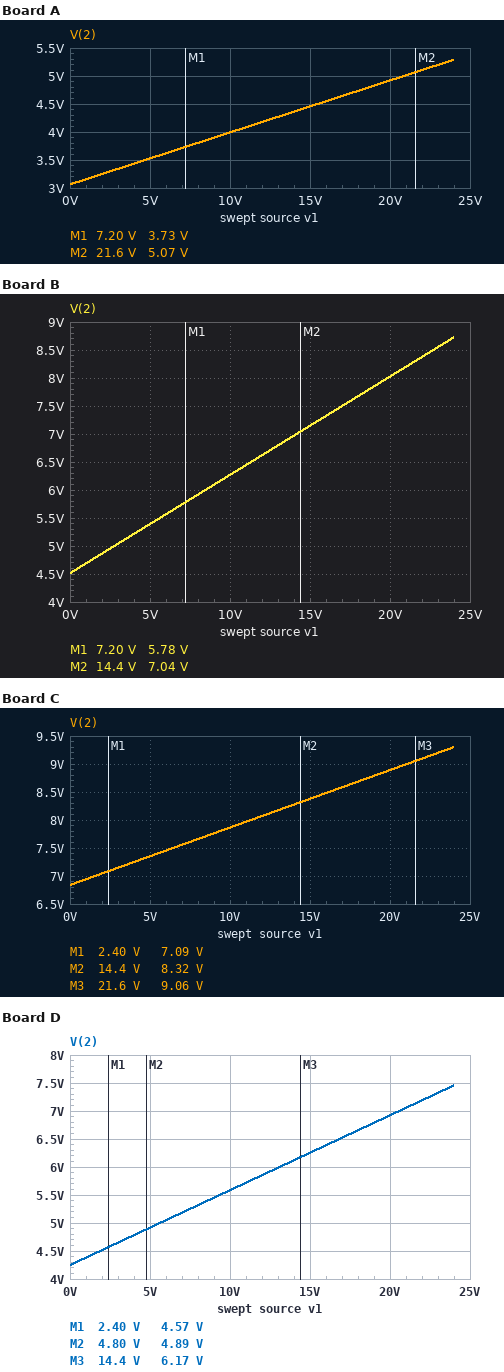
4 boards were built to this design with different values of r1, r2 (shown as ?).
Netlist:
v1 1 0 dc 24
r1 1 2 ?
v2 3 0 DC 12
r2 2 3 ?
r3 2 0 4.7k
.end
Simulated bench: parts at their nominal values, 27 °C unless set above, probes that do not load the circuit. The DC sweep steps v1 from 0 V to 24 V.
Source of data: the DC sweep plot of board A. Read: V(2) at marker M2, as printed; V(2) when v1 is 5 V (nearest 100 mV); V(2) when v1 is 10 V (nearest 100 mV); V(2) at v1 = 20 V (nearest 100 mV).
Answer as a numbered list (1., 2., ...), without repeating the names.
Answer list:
1. 5.07 V
2. 3.5 V
3. 4.0 V
4. 4.9 V
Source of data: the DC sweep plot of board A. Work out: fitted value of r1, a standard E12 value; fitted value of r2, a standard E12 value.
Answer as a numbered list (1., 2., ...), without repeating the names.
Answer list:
1. 33 kΩ
2. 12 kΩ
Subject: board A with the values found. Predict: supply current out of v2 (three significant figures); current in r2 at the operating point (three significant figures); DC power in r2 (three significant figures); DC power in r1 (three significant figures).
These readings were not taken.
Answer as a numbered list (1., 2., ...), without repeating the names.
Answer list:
1. 559 µA
2. 559 µA
3. 3.75 mW
4. 10.6 mW
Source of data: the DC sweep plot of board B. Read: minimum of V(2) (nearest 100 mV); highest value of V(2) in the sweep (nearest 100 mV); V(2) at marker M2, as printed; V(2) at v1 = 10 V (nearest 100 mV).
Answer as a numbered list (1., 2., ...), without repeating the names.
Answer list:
1. 4.5 V
2. 8.7 V
3. 7.04 V
4. 6.3 V
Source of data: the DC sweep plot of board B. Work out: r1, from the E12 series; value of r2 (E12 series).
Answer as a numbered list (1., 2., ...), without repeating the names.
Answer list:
1. 12 kΩ
2. 5.6 kΩ
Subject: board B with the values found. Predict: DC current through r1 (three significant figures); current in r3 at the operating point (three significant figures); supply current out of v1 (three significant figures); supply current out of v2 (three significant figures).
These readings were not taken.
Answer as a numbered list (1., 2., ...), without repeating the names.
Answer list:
1. 1.27 mA
2. 1.86 mA
3. 1.27 mA
4. 584 µA
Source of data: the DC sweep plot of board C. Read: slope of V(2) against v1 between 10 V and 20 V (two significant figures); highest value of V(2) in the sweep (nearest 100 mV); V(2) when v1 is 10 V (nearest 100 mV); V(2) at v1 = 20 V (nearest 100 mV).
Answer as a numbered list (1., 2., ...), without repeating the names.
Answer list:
1. 0.10 V/V
2. 9.3 V
3. 7.9 V
4. 8.9 V
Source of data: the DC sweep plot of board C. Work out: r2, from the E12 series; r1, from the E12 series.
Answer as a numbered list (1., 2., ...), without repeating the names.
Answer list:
1. 2.7 kΩ
2. 15 kΩ
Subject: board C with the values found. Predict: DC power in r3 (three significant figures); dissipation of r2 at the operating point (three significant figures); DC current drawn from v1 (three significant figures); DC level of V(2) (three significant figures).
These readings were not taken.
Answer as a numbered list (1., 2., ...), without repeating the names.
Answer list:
1. 18.4 mW
2. 2.70 mW
3. 980 µA
4. 9.30 V
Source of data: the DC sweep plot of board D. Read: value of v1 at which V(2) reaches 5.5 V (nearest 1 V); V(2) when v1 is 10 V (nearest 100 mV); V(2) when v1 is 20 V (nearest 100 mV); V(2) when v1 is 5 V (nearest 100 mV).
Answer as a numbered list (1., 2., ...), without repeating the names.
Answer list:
1. 9 V
2. 5.6 V
3. 6.9 V
4. 4.9 V
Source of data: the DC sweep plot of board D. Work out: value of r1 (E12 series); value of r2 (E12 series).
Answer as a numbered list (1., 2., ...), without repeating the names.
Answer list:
1. 18 kΩ
2. 6.8 kΩ
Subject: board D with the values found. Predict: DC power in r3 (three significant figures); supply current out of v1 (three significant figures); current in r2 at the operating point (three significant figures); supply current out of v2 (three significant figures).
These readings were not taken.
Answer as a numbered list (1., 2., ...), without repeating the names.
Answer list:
1. 11.8 mW
2. 919 µA
3. 668 µA
4. 668 µA
